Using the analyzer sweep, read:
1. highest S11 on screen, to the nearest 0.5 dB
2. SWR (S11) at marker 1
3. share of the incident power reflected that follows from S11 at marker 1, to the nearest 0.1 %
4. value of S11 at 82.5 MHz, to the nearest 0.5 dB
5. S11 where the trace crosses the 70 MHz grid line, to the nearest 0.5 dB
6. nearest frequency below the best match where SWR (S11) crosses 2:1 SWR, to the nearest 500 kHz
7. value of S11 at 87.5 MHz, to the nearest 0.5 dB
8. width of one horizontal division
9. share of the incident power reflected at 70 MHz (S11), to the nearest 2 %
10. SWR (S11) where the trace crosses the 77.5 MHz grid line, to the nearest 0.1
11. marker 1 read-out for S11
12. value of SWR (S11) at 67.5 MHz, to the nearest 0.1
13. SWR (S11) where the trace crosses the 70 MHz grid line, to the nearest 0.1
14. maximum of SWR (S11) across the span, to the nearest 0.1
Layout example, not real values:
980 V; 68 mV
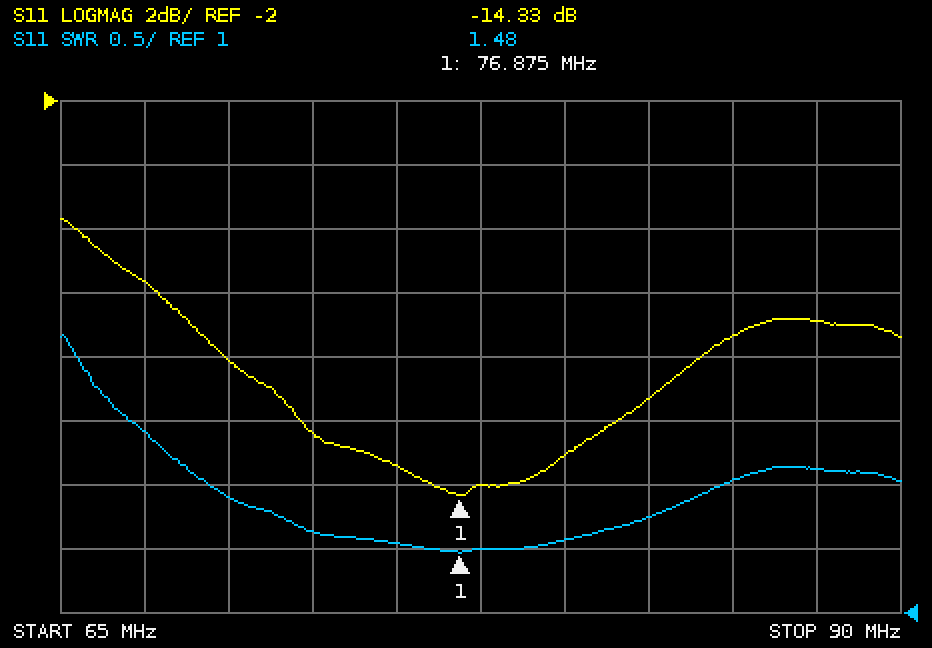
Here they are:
-5.5 dB; 1.48; 3.7 %; -11.5 dB; -10.0 dB; 69.5 MHz; -9.0 dB; 2.5 MHz; 10 %; 1.5; -14.33 dB; 2.4; 1.9; 3.2
